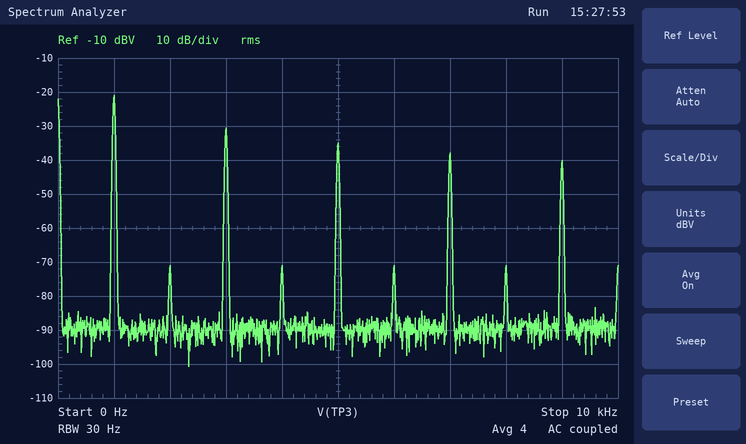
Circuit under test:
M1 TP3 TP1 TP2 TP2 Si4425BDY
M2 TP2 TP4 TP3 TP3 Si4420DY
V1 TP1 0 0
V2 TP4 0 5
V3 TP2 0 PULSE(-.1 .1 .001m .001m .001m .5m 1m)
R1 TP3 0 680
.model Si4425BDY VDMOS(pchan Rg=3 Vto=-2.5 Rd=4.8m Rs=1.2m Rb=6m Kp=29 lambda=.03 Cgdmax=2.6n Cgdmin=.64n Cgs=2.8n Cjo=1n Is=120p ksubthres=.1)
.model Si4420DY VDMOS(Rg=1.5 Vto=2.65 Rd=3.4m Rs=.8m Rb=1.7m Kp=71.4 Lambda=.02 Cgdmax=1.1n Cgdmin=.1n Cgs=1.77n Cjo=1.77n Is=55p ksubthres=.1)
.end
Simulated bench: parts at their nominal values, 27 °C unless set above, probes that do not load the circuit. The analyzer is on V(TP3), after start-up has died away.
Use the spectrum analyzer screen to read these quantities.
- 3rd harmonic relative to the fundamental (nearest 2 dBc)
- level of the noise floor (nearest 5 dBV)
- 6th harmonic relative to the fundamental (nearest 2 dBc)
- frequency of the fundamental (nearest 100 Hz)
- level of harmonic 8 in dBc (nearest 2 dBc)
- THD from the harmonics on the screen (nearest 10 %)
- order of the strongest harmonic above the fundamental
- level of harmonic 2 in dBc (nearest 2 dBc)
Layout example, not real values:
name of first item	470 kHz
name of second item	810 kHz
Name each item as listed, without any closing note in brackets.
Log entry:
3rd harmonic relative to the fundamental	-10 dBc
level of the noise floor	-90 dBV
6th harmonic relative to the fundamental	-50 dBc
frequency of the fundamental	1.0 kHz
level of harmonic 8 in dBc	-50 dBc
THD from the harmonics on the screen	40 %
order of the strongest harmonic above the fundamental	3
level of harmonic 2 in dBc	-50 dBc
